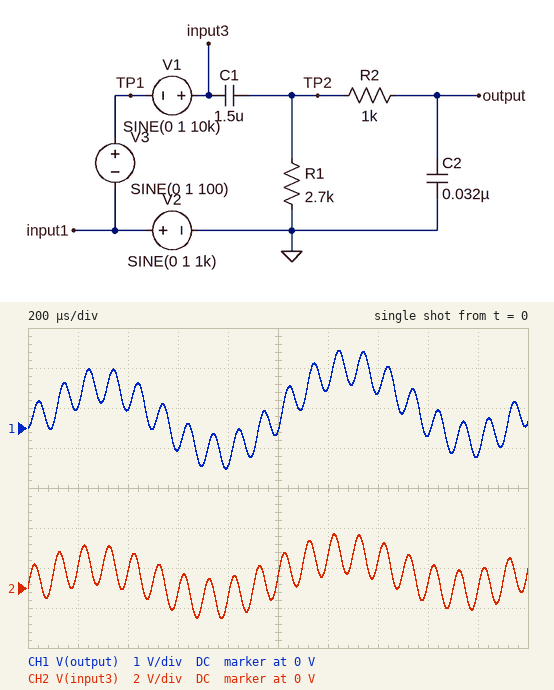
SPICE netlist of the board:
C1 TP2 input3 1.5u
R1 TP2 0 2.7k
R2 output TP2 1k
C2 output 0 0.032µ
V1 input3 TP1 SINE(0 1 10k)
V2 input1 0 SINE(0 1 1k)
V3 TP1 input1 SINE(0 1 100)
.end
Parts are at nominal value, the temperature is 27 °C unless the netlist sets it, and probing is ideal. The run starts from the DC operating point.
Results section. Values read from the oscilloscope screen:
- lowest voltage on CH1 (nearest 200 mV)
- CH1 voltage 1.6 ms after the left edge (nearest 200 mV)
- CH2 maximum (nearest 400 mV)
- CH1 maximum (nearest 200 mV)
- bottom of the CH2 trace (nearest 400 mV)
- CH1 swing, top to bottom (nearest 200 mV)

-1.0 V
-200 mV
2.8 V
2.0 V
-1.6 V
3.0 V
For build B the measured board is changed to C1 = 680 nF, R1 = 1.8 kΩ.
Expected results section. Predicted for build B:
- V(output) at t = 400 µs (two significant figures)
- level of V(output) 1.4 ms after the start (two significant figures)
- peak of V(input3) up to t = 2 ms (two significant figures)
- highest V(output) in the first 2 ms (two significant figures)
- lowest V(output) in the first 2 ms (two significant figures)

300 mV
590 mV
2.7 V
1.7 V
-1.1 V
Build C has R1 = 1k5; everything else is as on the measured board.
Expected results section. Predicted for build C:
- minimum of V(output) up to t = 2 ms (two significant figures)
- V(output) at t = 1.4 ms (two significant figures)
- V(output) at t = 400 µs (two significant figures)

-1.1 V
770 mV
410 mV
